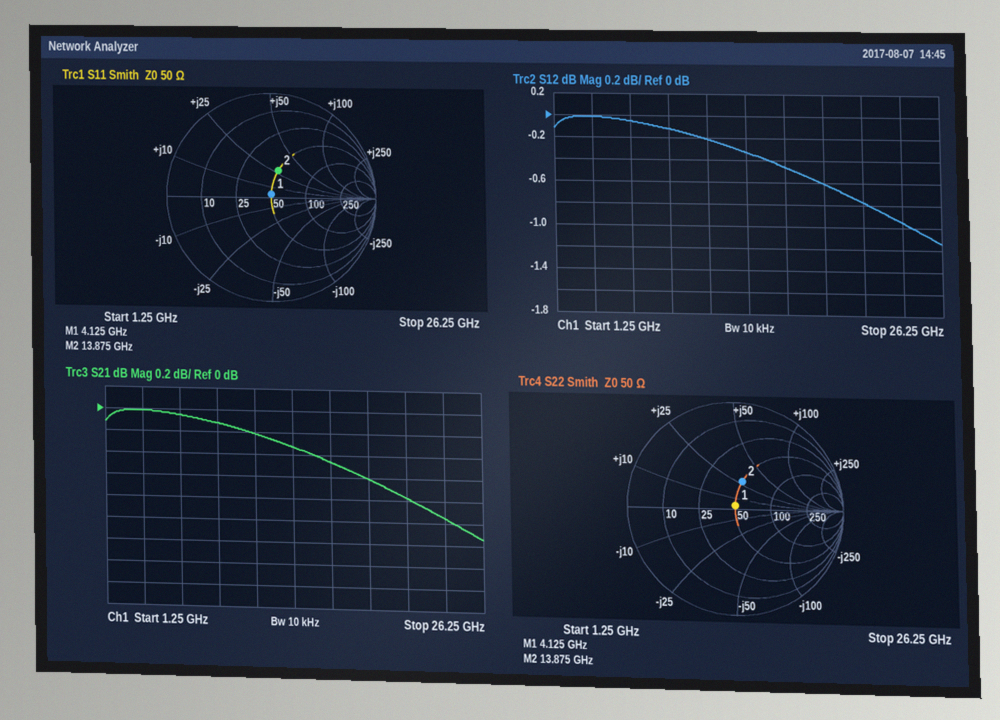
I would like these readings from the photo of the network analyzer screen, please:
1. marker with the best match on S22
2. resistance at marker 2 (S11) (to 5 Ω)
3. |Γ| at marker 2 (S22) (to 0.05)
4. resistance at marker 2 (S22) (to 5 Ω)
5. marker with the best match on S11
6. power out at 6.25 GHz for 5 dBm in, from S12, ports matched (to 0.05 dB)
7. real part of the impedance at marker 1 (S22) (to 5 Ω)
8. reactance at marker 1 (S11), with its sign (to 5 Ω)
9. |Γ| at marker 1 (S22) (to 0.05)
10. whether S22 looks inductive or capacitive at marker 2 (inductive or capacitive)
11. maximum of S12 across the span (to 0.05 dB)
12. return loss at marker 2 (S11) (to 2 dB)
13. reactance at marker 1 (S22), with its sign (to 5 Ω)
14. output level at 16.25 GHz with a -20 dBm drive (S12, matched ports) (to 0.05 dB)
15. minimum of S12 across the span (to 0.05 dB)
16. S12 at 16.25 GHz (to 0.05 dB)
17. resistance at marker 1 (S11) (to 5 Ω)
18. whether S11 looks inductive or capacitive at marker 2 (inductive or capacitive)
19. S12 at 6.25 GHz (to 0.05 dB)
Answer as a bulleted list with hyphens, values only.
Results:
- marker 1
- 50 Ω
- 0.25
- 50 Ω
- marker 1
- 4.95 dBm
- 50 Ω
- +5 Ω
- 0.05
- inductive
- 0.00 dB
- 12 dB
- +5 Ω
- -20.45 dBm
- -1.15 dB
- -0.45 dB
- 50 Ω
- inductive
- -0.05 dB
